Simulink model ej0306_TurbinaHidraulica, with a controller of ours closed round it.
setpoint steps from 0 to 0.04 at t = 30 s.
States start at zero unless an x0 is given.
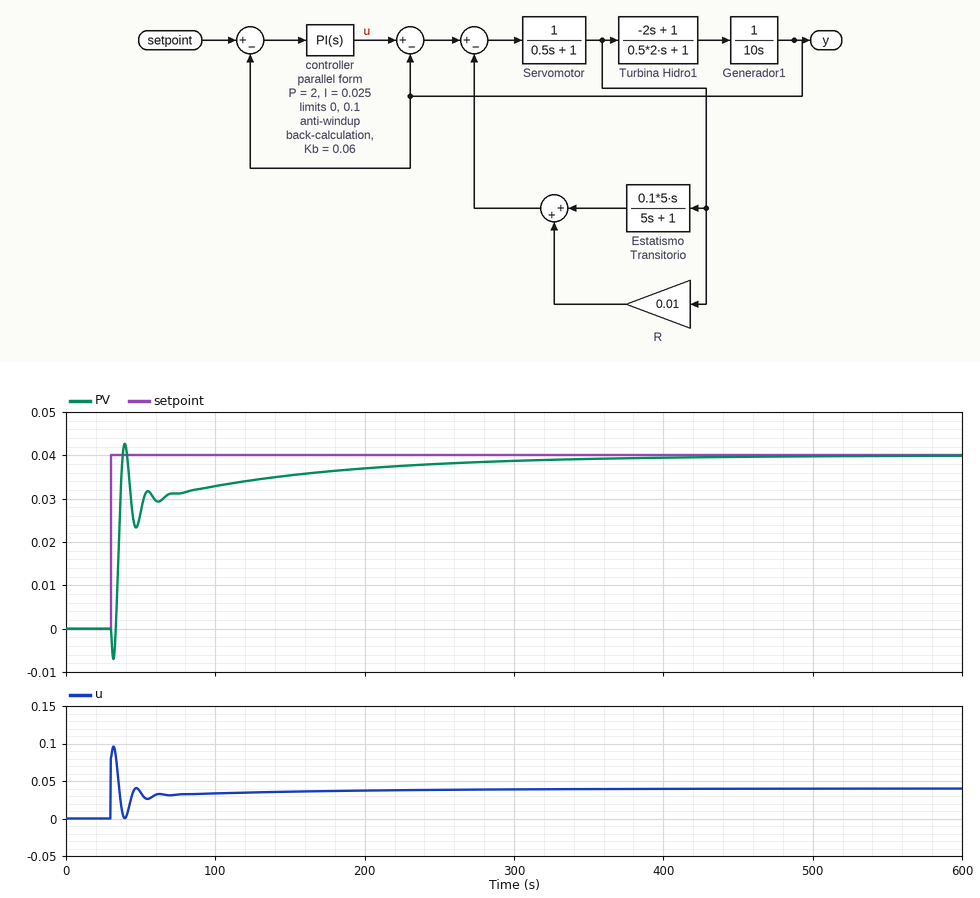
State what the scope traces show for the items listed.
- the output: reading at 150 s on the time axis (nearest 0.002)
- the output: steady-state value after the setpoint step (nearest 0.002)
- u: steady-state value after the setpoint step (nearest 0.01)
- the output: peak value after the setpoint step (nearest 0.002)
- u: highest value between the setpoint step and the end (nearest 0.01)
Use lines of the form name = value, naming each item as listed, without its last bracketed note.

the output: reading at 150 s on the time axis = 0.036
the output: steady-state value after the setpoint step = 0.040
u: steady-state value after the setpoint step = 0.04
the output: peak value after the setpoint step = 0.042
u: highest value between the setpoint step and the end = 0.10
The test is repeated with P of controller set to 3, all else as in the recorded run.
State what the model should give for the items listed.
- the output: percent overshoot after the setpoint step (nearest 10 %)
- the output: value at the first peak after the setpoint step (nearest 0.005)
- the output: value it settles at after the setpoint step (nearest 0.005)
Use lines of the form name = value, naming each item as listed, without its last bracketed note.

the output: percent overshoot after the setpoint step = 20 %
the output: value at the first peak after the setpoint step = 0.050
the output: value it settles at after the setpoint step = 0.040
